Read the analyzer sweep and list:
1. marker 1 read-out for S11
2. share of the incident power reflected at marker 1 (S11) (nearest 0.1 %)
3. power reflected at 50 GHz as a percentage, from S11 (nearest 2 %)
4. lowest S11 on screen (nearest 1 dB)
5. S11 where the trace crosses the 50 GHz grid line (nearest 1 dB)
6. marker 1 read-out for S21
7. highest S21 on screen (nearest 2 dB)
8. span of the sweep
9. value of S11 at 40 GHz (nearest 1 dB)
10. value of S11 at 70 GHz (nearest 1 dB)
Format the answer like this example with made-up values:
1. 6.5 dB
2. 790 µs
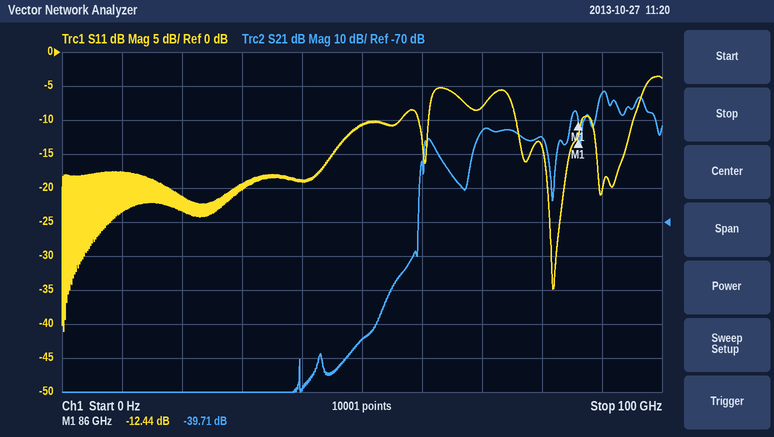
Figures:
1. -12.44 dB
2. 5.7 %
3. 8 %
4. -41 dB
5. -11 dB
6. -39.71 dB
7. -32 dB
8. 100 GHz
9. -19 dB
10. -8 dB
